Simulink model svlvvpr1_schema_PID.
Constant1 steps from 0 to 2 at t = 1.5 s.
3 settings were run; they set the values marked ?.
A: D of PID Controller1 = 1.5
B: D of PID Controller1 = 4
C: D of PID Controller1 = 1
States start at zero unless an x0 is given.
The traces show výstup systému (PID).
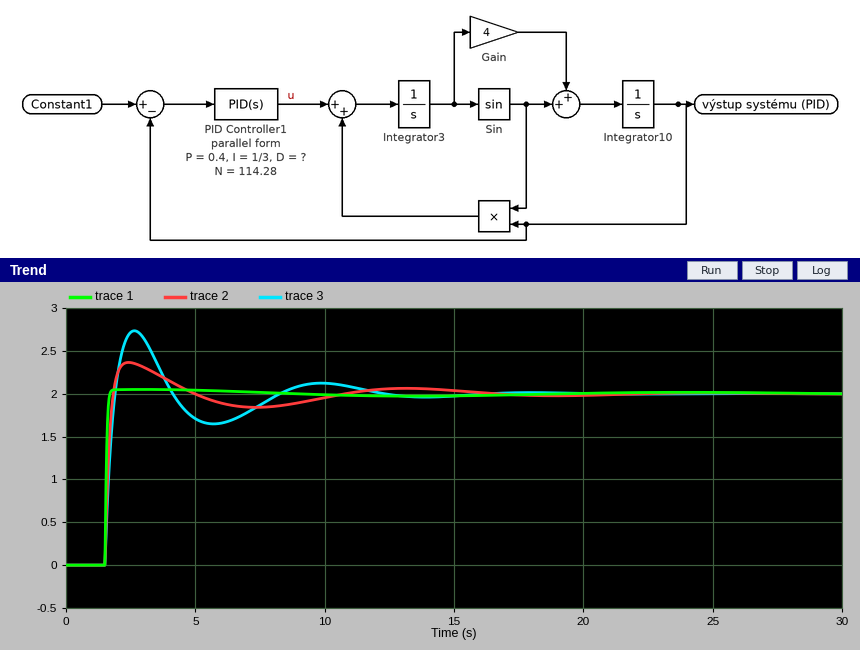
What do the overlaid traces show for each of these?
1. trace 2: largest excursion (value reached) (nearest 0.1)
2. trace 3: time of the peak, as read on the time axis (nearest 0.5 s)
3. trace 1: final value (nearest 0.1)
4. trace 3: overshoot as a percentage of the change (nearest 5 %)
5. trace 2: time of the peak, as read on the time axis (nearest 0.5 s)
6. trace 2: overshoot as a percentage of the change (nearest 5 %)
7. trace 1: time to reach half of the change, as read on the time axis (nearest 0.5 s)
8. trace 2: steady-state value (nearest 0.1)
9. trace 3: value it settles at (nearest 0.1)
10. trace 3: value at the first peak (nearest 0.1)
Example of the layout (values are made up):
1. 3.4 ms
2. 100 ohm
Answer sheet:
1. 2.4
2. 2.5 s
3. 2.0
4. 35 %
5. 2.5 s
6. 20 %
7. 1.5 s
8. 2.0
9. 2.0
10. 2.7
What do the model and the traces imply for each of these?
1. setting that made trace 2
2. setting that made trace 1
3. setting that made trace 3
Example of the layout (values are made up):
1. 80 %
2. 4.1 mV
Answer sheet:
1. A
2. B
3. C
